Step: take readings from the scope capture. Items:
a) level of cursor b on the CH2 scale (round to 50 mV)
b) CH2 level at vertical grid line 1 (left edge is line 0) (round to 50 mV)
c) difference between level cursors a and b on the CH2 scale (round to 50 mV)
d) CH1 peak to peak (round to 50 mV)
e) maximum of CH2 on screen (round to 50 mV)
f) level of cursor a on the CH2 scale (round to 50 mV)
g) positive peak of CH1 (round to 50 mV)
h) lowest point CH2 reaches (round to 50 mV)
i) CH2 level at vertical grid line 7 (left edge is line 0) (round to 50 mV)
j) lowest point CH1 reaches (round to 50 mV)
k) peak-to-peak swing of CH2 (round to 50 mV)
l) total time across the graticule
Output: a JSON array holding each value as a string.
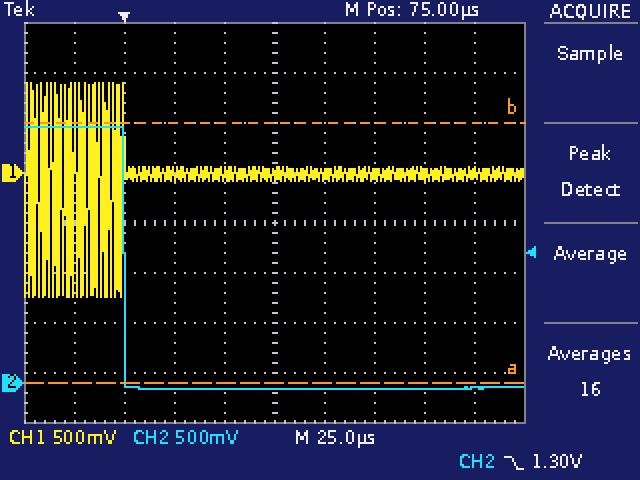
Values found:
["2.60 V", "2.55 V", "2.60 V", "2.15 V", "2.55 V", "0 mV", "900 mV", "-50 mV", "-50 mV", "-1.25 V", "2.60 V", "250 µs"]
